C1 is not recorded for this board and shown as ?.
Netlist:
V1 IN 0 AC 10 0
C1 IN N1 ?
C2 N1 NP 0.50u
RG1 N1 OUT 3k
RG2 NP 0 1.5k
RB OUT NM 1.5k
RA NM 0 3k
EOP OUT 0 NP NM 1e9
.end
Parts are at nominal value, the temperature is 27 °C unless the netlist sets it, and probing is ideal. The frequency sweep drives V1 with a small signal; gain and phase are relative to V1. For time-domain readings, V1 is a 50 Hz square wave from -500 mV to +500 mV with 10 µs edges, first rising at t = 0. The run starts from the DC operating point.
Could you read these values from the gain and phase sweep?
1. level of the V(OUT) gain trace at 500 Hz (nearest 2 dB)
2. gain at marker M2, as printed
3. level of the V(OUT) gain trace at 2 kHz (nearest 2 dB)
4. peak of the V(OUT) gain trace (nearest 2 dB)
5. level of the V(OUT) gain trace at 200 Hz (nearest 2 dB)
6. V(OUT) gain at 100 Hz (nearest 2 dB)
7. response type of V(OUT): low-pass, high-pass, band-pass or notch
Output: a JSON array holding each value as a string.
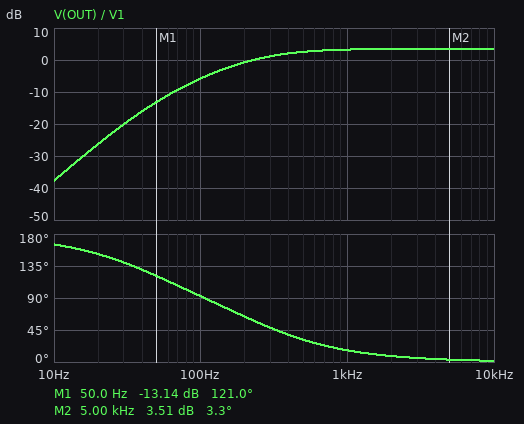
["2 dB", "3.51 dB", "4 dB", "4 dB", "0 dB", "-6 dB", "high-pass"]
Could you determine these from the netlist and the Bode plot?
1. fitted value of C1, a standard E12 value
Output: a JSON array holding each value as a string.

["1 µF"]
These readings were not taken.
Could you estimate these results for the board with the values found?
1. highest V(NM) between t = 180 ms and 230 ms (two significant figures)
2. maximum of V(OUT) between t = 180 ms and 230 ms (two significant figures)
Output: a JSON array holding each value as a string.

["1.0 V", "1.5 V"]
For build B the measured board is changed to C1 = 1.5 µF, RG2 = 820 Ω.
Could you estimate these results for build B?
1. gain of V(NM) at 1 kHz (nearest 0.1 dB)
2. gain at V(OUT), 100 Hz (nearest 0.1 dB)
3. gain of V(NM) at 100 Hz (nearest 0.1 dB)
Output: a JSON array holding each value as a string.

["-0.9 dB", "-10.5 dB", "-14.0 dB"]
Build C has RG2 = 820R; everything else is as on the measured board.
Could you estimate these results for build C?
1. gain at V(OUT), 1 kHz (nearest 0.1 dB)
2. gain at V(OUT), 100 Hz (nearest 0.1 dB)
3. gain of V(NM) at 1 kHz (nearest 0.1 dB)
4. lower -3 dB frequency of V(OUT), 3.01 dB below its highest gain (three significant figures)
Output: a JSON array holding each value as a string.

["2.5 dB", "-11.5 dB", "-1.0 dB", "519 Hz"]
